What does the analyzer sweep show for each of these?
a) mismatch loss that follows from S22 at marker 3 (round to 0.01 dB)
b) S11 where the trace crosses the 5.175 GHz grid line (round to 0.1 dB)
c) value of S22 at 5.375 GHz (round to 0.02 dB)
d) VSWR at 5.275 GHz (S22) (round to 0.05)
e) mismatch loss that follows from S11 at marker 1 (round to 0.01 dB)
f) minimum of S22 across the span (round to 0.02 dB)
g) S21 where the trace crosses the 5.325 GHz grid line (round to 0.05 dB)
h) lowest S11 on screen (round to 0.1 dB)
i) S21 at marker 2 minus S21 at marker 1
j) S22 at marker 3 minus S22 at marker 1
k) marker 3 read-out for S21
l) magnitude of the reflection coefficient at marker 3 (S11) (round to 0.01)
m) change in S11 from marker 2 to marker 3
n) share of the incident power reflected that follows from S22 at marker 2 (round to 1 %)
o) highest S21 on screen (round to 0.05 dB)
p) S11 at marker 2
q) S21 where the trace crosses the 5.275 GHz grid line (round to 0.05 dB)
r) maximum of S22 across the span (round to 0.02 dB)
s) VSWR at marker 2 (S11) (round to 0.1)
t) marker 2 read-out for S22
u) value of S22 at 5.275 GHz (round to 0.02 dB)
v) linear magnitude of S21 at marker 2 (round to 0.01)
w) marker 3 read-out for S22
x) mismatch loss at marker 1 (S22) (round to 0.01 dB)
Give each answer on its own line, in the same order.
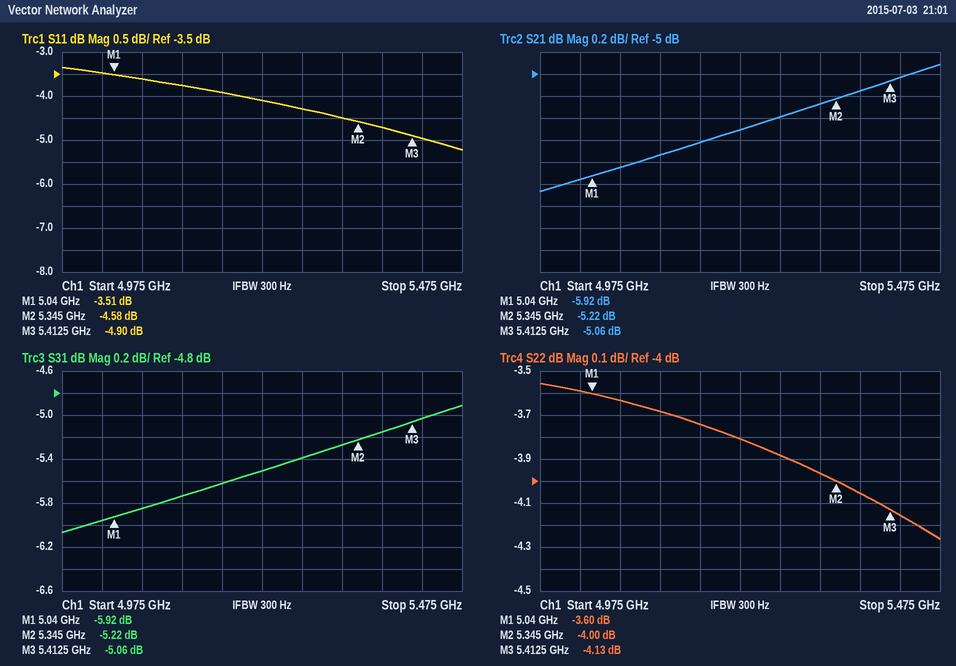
2.12 dB
-3.9 dB
-4.06 dB
4.55
2.56 dB
-4.26 dB
-5.25 dB
-5.2 dB
0.70 dB
-0.53 dB
-5.06 dB
0.57
-0.32 dB
40 %
-4.90 dB
-4.58 dB
-5.40 dB
-3.56 dB
3.9
-4.00 dB
-3.88 dB
0.55
-4.13 dB
2.49 dB
